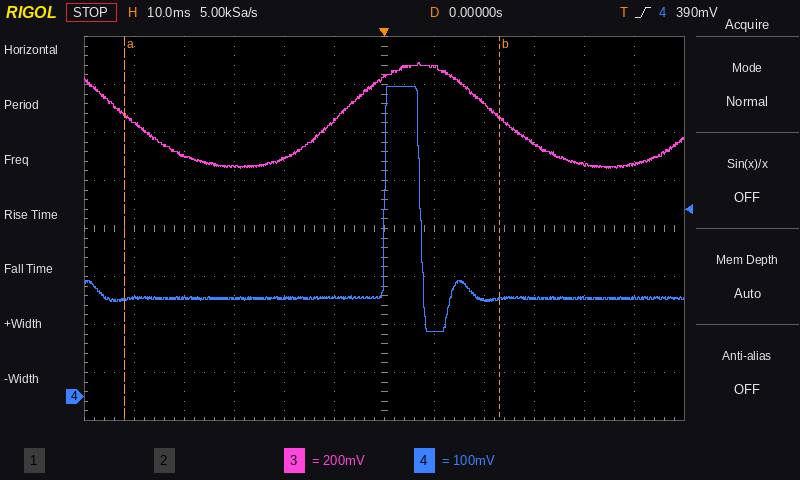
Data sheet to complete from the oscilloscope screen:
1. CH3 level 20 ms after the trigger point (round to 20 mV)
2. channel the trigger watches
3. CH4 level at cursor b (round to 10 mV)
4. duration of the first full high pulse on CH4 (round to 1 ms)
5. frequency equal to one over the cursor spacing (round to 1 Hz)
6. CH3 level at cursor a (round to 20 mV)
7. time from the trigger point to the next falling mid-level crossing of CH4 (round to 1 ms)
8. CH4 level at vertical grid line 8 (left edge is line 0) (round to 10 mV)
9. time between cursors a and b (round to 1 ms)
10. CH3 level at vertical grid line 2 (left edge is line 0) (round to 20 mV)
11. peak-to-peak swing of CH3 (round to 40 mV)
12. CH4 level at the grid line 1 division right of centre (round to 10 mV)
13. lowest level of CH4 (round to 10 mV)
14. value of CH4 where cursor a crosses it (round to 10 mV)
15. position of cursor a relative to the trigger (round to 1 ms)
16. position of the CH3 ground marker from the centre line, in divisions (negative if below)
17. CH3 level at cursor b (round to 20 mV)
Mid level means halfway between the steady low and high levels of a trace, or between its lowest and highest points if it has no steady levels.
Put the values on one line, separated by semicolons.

1.22 V; CH4; 200 mV; 7 ms; 13 Hz; 1.18 V; 7 ms; 200 mV; 75 ms; 1.00 V; 440 mV; 140 mV; 140 mV; 200 mV; -52 ms; -3.5 div; 1.16 V
